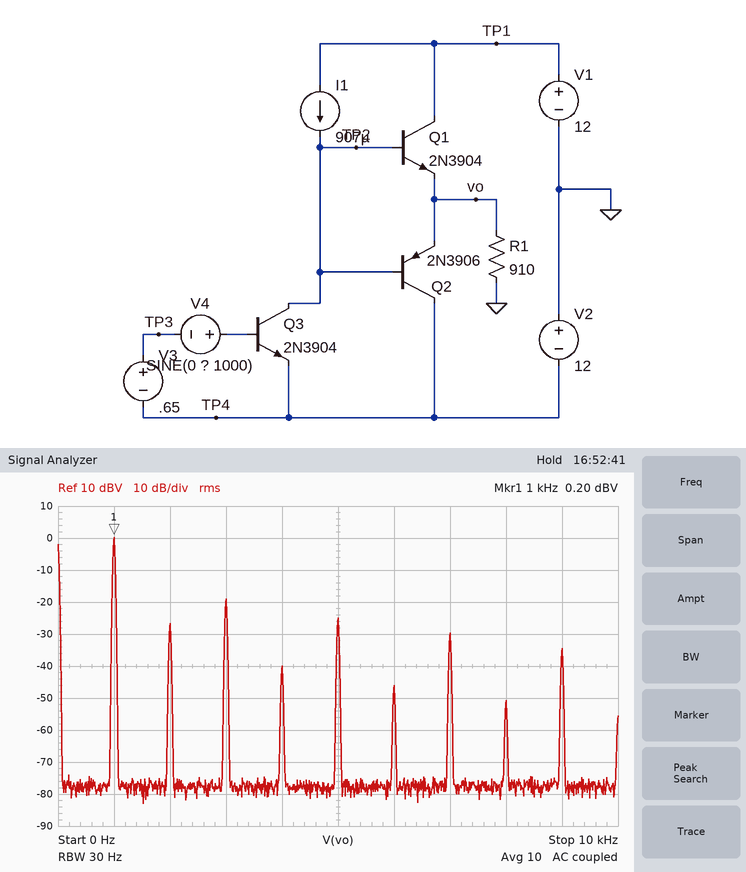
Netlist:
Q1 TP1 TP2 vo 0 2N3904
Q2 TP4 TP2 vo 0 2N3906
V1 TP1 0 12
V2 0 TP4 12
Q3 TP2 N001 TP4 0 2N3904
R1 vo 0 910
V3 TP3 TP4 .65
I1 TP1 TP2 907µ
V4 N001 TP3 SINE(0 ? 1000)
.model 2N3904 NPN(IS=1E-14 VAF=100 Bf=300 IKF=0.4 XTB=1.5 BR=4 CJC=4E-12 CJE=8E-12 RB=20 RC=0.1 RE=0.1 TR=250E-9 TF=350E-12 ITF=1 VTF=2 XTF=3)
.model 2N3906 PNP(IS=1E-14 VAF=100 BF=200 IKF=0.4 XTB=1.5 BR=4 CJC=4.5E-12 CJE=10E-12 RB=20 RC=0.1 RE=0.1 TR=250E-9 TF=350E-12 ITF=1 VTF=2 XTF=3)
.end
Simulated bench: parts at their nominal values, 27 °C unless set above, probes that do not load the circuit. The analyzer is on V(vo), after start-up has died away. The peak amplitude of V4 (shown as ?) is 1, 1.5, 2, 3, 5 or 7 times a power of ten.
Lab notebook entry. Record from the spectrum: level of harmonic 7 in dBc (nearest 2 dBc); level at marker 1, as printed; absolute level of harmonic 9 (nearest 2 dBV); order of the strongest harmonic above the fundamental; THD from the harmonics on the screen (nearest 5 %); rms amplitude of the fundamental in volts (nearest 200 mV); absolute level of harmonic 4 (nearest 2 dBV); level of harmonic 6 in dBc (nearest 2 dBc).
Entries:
-30 dBc
0.20 dBV
-34 dBV
3
15 %
1.0 V
-40 dBV
-46 dBc
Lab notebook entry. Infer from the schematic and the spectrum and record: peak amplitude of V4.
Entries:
700 µV
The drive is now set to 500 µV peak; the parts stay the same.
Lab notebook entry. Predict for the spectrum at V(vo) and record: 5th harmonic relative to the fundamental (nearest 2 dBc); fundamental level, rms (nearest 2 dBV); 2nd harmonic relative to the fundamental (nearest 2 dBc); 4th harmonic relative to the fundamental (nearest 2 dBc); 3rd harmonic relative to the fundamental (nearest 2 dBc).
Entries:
-22 dBc
-4 dBV
-26 dBc
-38 dBc
-16 dBc
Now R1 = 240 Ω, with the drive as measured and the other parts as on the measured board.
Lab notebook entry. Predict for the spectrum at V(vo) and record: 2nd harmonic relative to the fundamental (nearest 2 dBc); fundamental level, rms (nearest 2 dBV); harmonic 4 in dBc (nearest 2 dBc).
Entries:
-22 dBc
-6 dBV
-36 dBc
